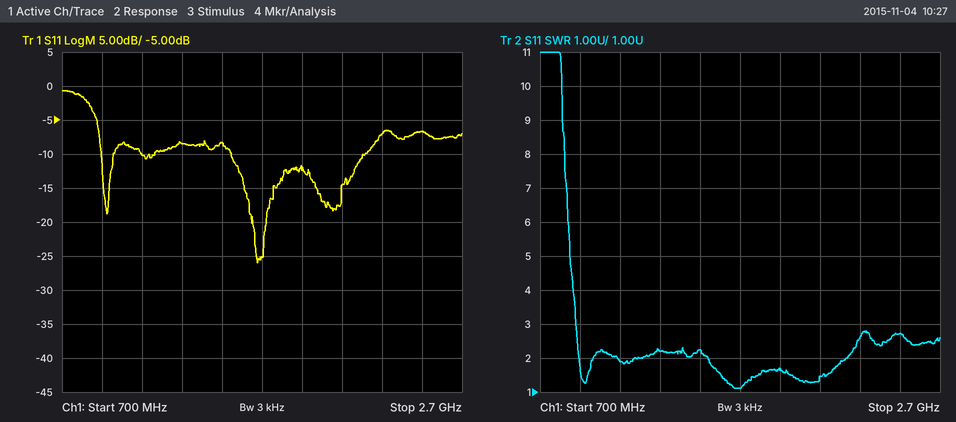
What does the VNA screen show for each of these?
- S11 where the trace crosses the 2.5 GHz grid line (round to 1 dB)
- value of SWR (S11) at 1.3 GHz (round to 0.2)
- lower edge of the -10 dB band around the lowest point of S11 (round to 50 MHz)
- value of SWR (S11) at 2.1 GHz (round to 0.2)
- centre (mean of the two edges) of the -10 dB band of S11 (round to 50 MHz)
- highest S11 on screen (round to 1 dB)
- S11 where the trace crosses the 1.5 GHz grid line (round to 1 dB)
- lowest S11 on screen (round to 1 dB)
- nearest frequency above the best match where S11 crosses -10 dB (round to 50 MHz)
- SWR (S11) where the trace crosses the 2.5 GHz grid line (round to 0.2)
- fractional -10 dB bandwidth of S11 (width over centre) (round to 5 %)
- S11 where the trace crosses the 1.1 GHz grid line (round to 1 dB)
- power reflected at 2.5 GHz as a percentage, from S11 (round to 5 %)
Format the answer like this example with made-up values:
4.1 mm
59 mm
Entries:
-7 dB
2.2
1.55 GHz
1.4
1.90 GHz
-1 dB
-8 dB
-26 dB
2.20 GHz
2.8
35 %
-10 dB
20 %
